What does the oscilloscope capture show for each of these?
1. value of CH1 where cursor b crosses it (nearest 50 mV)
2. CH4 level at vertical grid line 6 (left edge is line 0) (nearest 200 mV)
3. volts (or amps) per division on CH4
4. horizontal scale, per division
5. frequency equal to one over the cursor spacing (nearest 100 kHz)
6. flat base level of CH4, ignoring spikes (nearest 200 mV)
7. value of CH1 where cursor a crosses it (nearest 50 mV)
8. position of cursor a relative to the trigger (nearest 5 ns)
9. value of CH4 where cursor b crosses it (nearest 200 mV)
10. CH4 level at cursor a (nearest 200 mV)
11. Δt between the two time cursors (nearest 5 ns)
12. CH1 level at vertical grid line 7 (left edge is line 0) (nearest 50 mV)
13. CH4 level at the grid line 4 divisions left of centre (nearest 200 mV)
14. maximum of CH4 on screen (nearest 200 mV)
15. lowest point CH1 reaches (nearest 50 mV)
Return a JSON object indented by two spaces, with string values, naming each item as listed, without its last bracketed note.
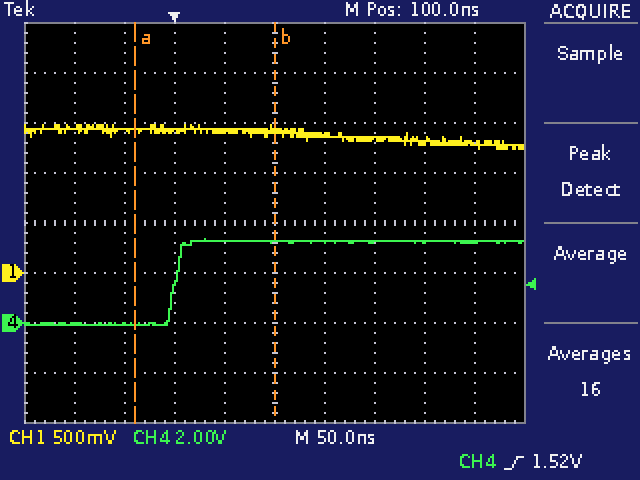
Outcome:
{
  "value of CH1 where cursor b crosses it": "1.45 V",
  "CH4 level at vertical grid line 6 (left edge is line 0)": "3.2 V",
  "volts (or amps) per division on CH4": "2 V",
  "horizontal scale, per division": "50 ns",
  "frequency equal to one over the cursor spacing": "7.1 MHz",
  "flat base level of CH4, ignoring spikes": "0.0 V",
  "value of CH1 where cursor a crosses it": "1.40 V",
  "position of cursor a relative to the trigger": "-40 ns",
  "value of CH4 where cursor b crosses it": "3.2 V",
  "CH4 level at cursor a": "0.0 V",
  "Δt between the two time cursors": "140 ns",
  "CH1 level at vertical grid line 7 (left edge is line 0)": "1.35 V",
  "CH4 level at the grid line 4 divisions left of centre": "0.0 V",
  "maximum of CH4 on screen": "3.4 V",
  "lowest point CH1 reaches": "1.25 V"
}
